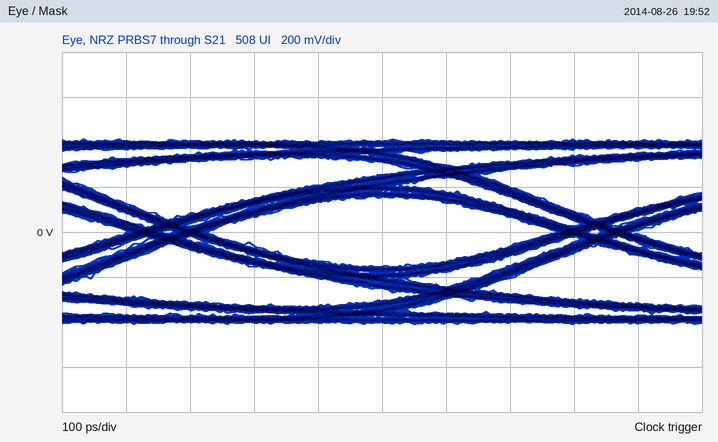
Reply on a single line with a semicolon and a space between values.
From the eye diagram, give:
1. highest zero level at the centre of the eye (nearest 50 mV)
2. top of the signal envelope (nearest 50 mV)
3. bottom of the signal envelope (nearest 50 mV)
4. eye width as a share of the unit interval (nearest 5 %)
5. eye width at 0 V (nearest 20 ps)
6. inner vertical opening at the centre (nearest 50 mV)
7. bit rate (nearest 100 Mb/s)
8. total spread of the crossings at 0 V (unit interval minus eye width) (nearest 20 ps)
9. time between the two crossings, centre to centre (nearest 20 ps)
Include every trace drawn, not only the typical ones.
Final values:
-150 mV; 400 mV; -400 mV; 80 %; 540 ps; 300 mV; 1.5 Gb/s; 120 ps; 660 ps
